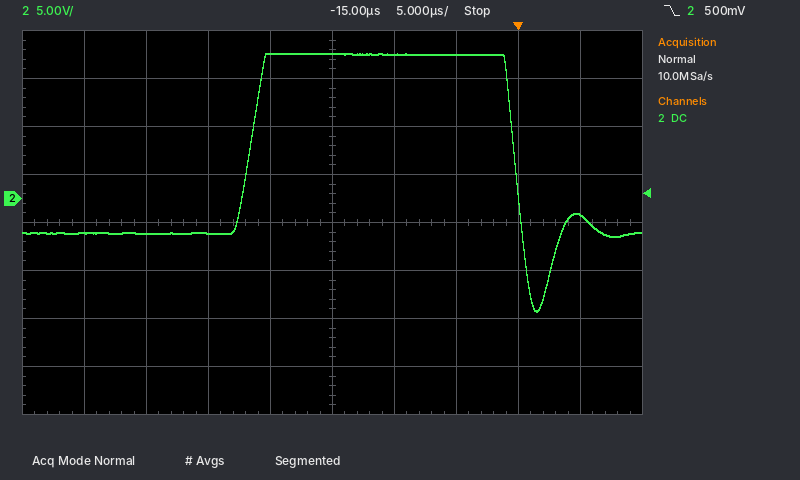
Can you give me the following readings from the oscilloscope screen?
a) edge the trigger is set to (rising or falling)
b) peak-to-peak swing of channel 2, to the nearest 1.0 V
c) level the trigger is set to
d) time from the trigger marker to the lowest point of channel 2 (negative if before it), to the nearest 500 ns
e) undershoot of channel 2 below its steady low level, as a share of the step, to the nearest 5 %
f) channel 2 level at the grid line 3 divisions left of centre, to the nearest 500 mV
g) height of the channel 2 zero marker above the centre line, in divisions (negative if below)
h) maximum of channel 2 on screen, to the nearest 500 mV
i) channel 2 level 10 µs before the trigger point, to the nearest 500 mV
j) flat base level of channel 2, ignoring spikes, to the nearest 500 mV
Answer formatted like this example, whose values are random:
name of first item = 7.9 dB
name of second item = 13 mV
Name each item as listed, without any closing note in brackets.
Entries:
edge the trigger is set to = falling
peak-to-peak swing of channel 2, to the nearest 1.0 V = 27.0 V
level the trigger is set to = 500 mV
time from the trigger marker to the lowest point of channel 2 (negative if before it), to the nearest 500 ns = +1.5 µs
undershoot of channel 2 below its steady low level, as a share of the step, to the nearest 5 % = 45 %
channel 2 level at the grid line 3 divisions left of centre, to the nearest 500 mV = -3.5 V
height of the channel 2 zero marker above the centre line, in divisions = +0.5 div
maximum of channel 2 on screen, to the nearest 500 mV = 15.0 V
channel 2 level 10 µs before the trigger point, to the nearest 500 mV = 15.0 V
flat base level of channel 2, ignoring spikes, to the nearest 500 mV = -3.5 V
